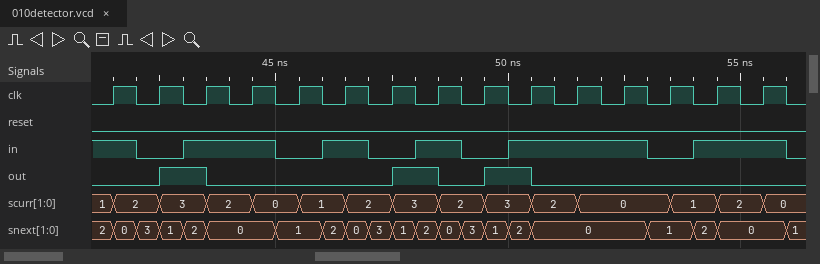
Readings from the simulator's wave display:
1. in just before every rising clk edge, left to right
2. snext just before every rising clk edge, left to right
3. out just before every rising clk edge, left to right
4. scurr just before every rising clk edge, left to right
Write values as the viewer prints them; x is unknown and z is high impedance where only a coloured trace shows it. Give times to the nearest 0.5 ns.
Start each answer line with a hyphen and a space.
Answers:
- 1 0 1 1 0 1 0 1 0 1 1 1 0 1 1
- 2, 3, 2, 0, 1, 2, 3, 2, 3, 2, 0, 0, 1, 2, 0
- 0 0 1 0 0 0 0 1 0 1 0 0 0 0 0
- 1, 2, 3, 2, 0, 1, 2, 3, 2, 3, 2, 0, 0, 1, 2
